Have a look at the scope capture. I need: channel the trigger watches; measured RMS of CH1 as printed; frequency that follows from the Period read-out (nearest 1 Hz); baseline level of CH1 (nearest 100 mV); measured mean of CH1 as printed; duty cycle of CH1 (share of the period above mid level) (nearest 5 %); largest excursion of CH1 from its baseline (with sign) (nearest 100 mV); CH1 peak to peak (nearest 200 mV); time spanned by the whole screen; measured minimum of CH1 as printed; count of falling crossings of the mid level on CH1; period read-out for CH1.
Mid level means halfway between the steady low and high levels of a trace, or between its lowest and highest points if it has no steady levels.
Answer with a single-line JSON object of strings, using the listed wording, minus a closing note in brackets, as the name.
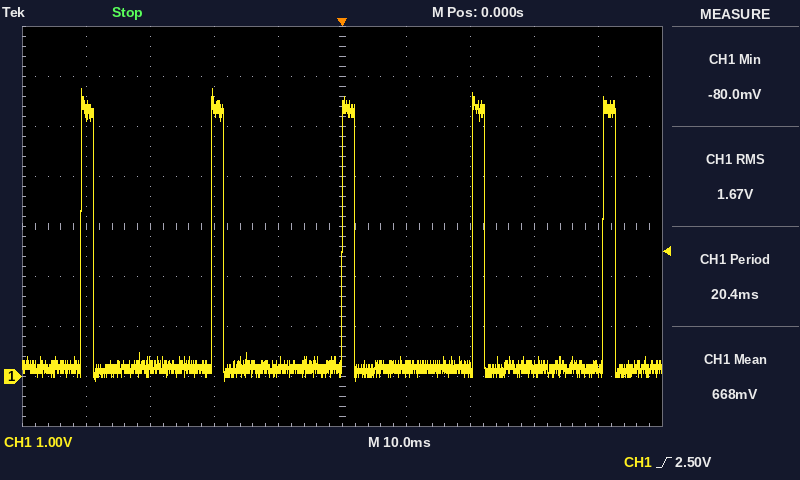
{"channel the trigger watches": "CH1", "measured RMS of CH1 as printed": "1.67 V", "frequency that follows from the Period read-out": "49 Hz", "baseline level of CH1": "200 mV", "measured mean of CH1 as printed": "668 mV", "duty cycle of CH1 (share of the period above mid level)": "10 %", "largest excursion of CH1 from its baseline (with sign)": "+5.6 V", "CH1 peak to peak": "5.8 V", "time spanned by the whole screen": "100 ms", "measured minimum of CH1 as printed": "-80.0 mV", "count of falling crossings of the mid level on CH1": "5", "period read-out for CH1": "20.4 ms"}
